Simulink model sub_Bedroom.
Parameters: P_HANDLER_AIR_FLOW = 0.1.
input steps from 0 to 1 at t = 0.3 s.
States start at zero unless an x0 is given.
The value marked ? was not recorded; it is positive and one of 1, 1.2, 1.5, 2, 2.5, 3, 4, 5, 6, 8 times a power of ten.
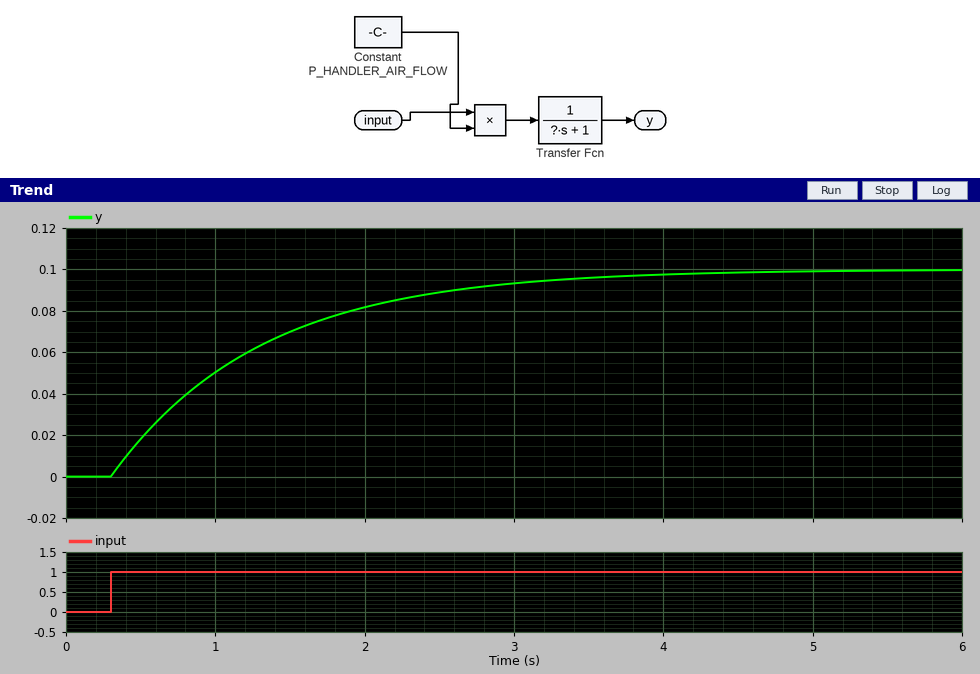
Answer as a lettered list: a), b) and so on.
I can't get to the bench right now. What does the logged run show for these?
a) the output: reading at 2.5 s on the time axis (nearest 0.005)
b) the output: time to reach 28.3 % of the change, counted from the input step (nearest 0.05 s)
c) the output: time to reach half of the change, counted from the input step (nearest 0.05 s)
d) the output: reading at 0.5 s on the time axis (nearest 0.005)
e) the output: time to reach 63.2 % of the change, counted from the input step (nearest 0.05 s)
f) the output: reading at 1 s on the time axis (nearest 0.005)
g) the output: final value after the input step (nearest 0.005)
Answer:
a) 0.090
b) 0.35 s
c) 0.70 s
d) 0.020
e) 1.00 s
f) 0.050
g) 0.100
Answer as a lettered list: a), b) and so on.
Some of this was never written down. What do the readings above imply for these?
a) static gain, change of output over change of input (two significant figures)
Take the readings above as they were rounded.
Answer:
a) 0.10
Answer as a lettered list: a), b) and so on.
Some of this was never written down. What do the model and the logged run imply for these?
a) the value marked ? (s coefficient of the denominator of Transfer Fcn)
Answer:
a) 1
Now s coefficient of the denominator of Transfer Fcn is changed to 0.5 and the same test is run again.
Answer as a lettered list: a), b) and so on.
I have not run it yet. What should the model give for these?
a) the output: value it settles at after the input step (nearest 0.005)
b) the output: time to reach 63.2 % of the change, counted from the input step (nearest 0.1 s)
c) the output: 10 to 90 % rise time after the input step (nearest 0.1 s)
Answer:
a) 0.100
b) 0.5 s
c) 1.1 s
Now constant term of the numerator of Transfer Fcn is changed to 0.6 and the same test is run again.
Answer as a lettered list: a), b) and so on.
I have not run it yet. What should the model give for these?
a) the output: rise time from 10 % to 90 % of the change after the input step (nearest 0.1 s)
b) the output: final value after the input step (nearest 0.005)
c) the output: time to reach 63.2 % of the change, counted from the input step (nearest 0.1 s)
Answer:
a) 2.2 s
b) 0.060
c) 1.0 s
